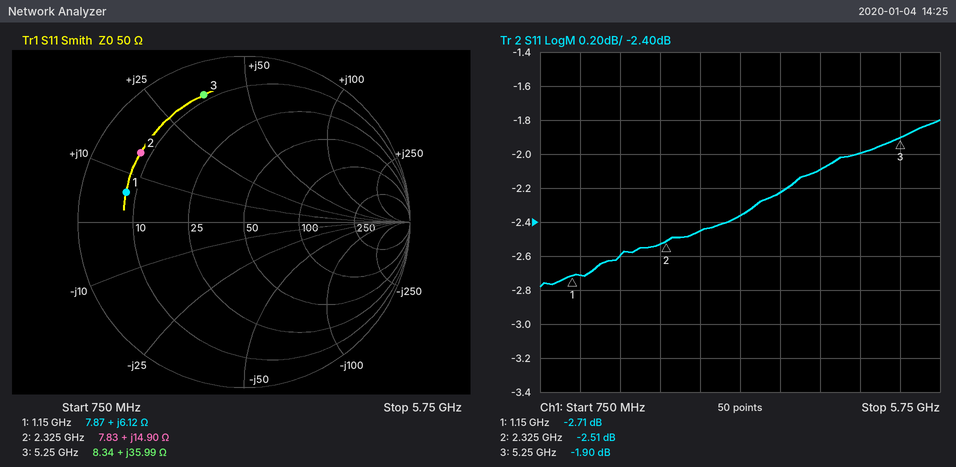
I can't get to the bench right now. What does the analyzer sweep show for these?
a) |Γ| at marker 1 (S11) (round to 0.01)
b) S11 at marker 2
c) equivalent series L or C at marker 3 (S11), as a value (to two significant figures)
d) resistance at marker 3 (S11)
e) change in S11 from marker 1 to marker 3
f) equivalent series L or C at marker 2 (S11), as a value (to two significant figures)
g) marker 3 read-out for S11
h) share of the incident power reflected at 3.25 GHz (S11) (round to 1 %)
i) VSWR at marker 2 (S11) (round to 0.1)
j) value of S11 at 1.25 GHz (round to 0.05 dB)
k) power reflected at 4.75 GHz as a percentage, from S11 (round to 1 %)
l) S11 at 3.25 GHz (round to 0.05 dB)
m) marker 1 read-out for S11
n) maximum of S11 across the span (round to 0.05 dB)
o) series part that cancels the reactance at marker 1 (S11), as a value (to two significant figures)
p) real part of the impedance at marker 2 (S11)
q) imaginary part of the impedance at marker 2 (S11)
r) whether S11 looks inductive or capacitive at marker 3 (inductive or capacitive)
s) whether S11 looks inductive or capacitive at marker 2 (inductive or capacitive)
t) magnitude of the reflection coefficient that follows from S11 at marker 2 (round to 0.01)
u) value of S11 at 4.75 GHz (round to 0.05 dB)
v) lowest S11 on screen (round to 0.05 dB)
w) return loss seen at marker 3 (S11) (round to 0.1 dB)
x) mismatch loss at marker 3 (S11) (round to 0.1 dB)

0.73
-2.51 dB
1.1 nH
8.34 Ω
0.81 dB
1.0 nH
-1.90 dB
58 %
7.0
-2.70 dB
63 %
-2.35 dB
-2.71 dB
-1.80 dB
23 pF
7.83 Ω
+14.90 Ω
inductive
inductive
0.75
-2.00 dB
-2.80 dB
1.9 dB
4.5 dB
